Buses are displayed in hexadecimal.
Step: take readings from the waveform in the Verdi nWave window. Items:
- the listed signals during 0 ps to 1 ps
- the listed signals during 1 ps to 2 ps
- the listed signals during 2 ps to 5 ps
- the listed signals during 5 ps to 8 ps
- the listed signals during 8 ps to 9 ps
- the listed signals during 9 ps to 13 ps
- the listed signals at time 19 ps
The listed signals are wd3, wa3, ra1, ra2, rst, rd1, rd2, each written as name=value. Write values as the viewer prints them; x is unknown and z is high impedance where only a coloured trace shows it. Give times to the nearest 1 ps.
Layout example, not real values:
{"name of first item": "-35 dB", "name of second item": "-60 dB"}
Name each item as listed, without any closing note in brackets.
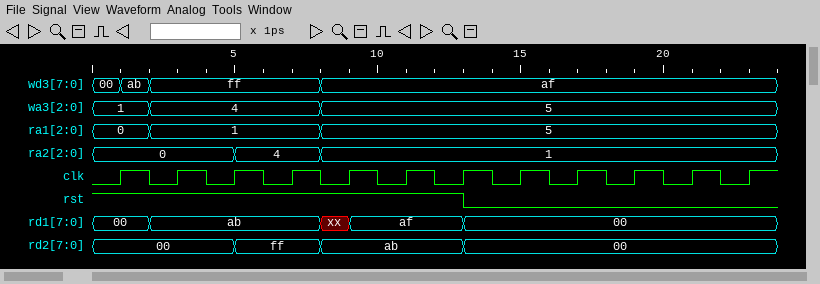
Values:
{"the listed signals during 0 ps to 1 ps": "wd3=00, wa3=1, ra1=0, ra2=0, rst=1, rd1=00, rd2=00", "the listed signals during 1 ps to 2 ps": "wd3=ab, wa3=1, ra1=0, ra2=0, rst=1, rd1=00, rd2=00", "the listed signals during 2 ps to 5 ps": "wd3=ff, wa3=4, ra1=1, ra2=0, rst=1, rd1=ab, rd2=00", "the listed signals during 5 ps to 8 ps": "wd3=ff, wa3=4, ra1=1, ra2=4, rst=1, rd1=ab, rd2=ff", "the listed signals during 8 ps to 9 ps": "wd3=af, wa3=5, ra1=5, ra2=1, rst=1, rd1=xx, rd2=ab", "the listed signals during 9 ps to 13 ps": "wd3=af, wa3=5, ra1=5, ra2=1, rst=1, rd1=af, rd2=ab", "the listed signals at time 19 ps": "wd3=af, wa3=5, ra1=5, ra2=1, rst=0, rd1=00, rd2=00"}
